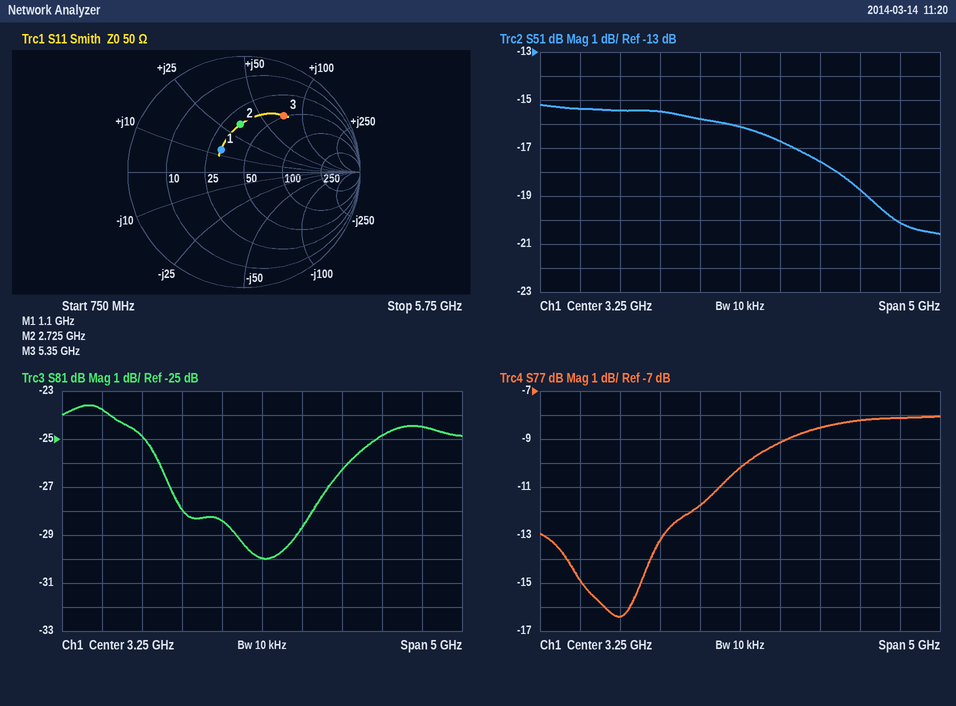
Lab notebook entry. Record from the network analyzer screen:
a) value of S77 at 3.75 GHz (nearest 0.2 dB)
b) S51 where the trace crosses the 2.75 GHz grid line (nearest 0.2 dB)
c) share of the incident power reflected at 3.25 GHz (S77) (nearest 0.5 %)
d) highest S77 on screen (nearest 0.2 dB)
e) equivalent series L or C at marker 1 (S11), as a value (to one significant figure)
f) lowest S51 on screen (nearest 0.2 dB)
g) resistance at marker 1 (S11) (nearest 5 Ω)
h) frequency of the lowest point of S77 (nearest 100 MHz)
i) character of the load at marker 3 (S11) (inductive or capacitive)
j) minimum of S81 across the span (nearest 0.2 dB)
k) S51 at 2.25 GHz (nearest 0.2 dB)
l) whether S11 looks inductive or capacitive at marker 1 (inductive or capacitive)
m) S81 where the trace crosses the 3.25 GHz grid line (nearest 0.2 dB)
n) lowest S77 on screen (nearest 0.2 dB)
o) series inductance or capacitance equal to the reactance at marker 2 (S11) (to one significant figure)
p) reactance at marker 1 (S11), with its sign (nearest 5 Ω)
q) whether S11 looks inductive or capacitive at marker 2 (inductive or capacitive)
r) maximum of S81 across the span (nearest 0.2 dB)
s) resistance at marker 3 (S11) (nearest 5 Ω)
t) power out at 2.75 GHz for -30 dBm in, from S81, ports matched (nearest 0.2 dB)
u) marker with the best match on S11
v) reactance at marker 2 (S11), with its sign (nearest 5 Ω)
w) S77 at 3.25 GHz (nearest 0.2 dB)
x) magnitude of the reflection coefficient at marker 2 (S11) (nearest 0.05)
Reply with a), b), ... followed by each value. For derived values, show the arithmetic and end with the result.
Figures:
a) -9.2 dB
b) -15.8 dB
c) 10^(-10.2/10) ≈ 9.5 %
d) -8.0 dB
e) L = 15 Ω/(2π × 1.1 GHz) ≈ 2 nH
f) -20.6 dB
g) 30 Ω
h) 1.7 GHz
i) inductive
j) -30.0 dB
k) -15.4 dB
l) inductive
m) -30.0 dB
n) -16.4 dB
o) L = 35 Ω/(2π × 2.725 GHz) ≈ 2 nH
p) +15 Ω
q) inductive
r) -23.6 dB
s) 50 Ω
t) -30 dBm + (-28.4 dB) = -58.4 dBm
u) marker 1
v) +35 Ω
w) -10.2 dB
x) 0.40
